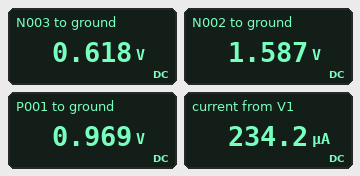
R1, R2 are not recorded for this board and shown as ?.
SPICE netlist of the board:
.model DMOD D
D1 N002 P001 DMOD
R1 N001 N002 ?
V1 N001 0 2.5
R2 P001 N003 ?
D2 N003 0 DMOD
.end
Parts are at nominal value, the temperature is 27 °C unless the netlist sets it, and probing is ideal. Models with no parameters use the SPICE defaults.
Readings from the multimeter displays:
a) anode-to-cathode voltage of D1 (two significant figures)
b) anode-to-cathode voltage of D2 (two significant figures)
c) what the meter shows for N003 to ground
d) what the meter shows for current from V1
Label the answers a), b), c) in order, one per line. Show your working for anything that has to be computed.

a) 1.587 V - 969 mV = 620 mV
b) 618 mV = 620 mV
c) 0.618 V
d) 234.2 µA
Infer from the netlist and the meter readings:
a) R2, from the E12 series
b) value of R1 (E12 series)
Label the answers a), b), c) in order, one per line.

a) 1.5 kΩ
b) 3.9 kΩ
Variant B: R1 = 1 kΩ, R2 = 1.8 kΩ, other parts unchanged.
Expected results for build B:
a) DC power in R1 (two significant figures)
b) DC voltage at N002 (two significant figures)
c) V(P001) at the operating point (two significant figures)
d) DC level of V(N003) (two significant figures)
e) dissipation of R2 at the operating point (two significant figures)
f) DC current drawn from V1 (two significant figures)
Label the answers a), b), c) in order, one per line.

a) 190 µW
b) 2.1 V
c) 1.4 V
d) 630 mV
e) 350 µW
f) 440 µA
